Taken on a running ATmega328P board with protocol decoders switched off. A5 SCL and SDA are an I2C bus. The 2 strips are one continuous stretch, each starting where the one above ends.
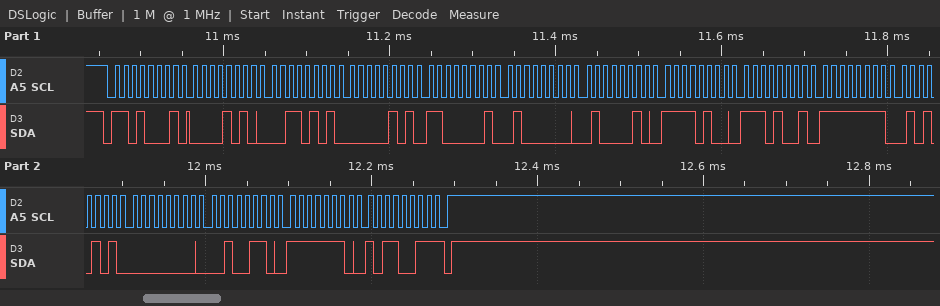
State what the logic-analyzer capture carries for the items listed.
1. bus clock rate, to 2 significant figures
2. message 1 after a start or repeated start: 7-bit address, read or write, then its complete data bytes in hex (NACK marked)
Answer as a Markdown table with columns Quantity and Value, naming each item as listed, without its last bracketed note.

| Quantity | Value |
|---|---|
| bus clock rate, to 2 significant figures | 100 kHz |
| message 1 after a start or repeated start: 7-bit address, read or write, then its complete data bytes in hex | 0x68 read: 0A 35 05 C1 40 42 F4 E9 FF 55 00 26 FE B3 NACK |
